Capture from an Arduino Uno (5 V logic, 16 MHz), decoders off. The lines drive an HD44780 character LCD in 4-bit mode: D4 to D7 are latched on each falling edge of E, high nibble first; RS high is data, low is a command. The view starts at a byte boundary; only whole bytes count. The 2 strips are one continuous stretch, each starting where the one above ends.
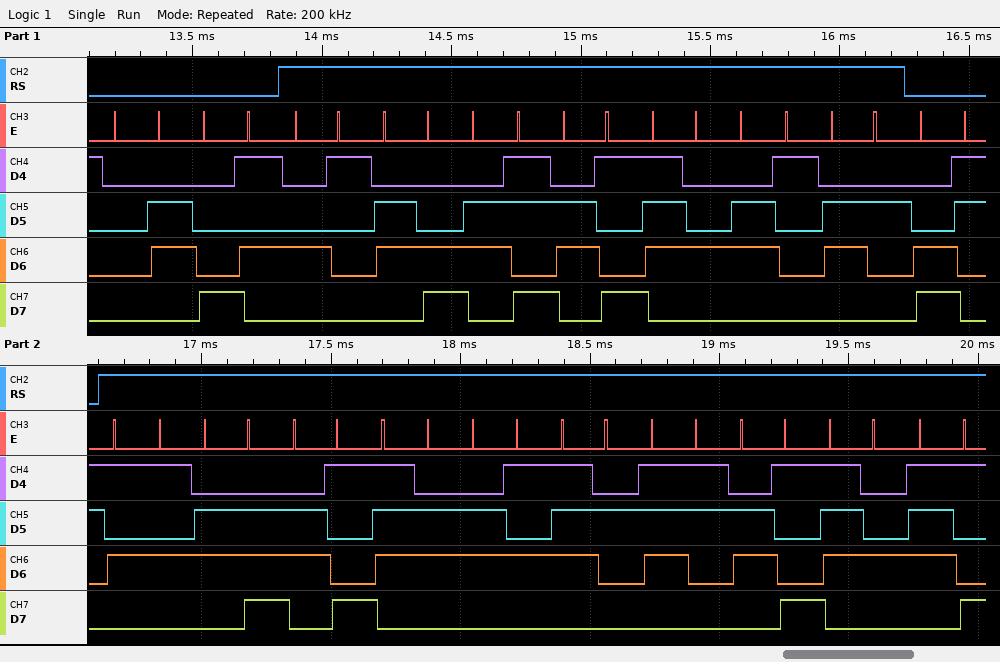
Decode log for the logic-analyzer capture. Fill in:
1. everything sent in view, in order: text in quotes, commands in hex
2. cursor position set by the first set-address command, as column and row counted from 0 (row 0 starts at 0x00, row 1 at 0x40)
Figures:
0x06 0x85 "Alkitab" 0xC3 "University"
column 5, row 0
